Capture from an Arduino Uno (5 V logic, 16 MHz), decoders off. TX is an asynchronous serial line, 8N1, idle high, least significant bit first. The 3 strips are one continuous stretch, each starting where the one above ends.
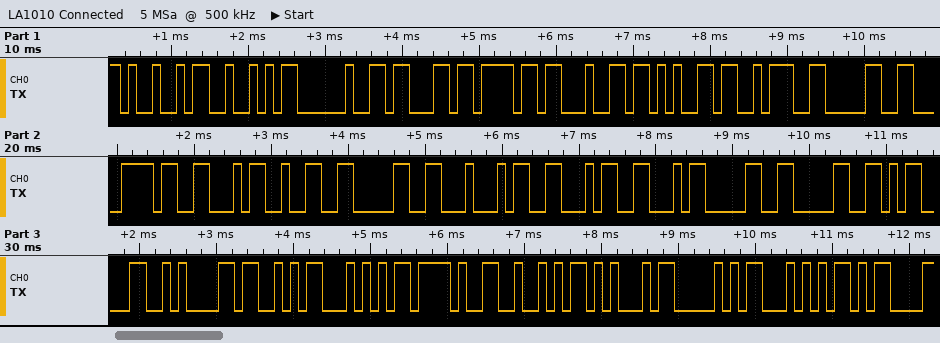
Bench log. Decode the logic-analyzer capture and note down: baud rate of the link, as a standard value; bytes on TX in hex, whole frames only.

9600 baud
0x49 0x52 0x20 0x63 0x6F 0x64 0x65 0x3A 0x30 0x78 0x46 0x32 0x30 0x44 0x46 0x46 0x30 0x30 0x0D 0x0A 0x53 0x54 0x2F 0x52 0x45 0x50 0x54 0x0D
